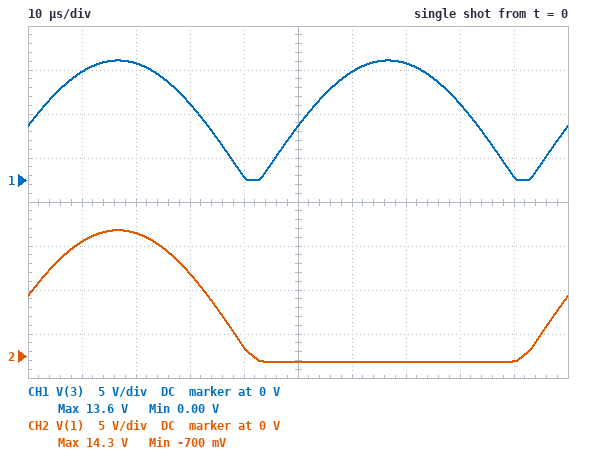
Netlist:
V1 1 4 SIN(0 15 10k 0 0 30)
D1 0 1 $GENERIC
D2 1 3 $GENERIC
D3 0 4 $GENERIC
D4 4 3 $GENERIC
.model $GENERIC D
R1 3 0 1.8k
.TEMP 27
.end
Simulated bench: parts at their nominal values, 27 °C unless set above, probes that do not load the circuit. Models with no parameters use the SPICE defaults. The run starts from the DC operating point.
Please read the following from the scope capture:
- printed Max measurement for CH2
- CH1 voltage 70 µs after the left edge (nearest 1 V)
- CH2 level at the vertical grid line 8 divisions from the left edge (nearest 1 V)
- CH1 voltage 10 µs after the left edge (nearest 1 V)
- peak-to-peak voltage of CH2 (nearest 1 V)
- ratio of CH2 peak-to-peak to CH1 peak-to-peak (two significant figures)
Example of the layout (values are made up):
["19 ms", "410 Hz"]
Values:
["14.3 V", "13 V", "-1 V", "12 V", "15 V", "1.1"]
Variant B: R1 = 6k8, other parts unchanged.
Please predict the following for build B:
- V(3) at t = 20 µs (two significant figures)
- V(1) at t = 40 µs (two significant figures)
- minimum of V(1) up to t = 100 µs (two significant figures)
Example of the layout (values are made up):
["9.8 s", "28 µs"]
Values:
["13 V", "990 mV", "-670 mV"]
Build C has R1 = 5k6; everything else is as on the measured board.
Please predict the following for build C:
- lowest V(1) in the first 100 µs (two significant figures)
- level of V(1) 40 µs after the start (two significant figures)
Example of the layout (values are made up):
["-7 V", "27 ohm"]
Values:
["-680 mV", "980 mV"]
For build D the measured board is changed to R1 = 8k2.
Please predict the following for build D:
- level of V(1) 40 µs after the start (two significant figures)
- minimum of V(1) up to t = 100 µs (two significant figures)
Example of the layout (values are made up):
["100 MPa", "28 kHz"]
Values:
["990 mV", "-670 mV"]
